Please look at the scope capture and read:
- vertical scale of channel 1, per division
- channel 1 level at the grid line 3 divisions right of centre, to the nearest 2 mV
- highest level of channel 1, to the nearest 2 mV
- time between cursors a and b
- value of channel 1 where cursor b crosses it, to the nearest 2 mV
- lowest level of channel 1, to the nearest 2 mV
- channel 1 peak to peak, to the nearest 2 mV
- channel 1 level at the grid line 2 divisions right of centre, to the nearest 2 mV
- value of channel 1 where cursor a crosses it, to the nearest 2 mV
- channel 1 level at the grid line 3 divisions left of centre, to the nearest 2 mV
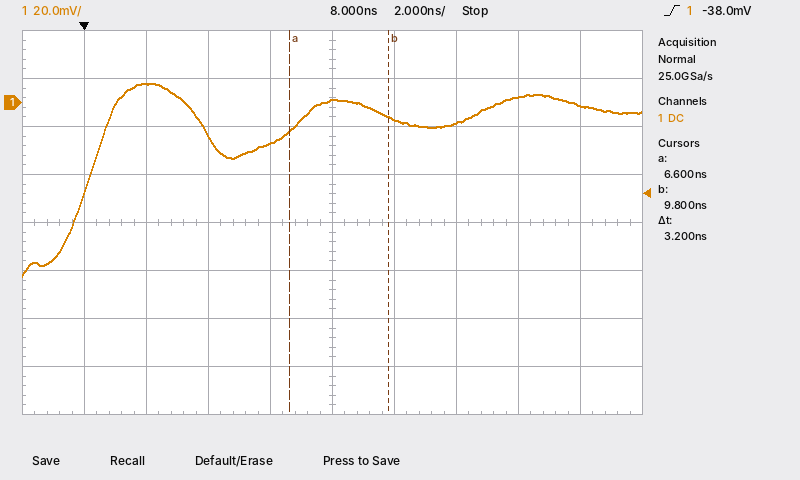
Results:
20 mV
2 mV
8 mV
3.2 ns
-6 mV
-72 mV
80 mV
-8 mV
-12 mV
8 mV
